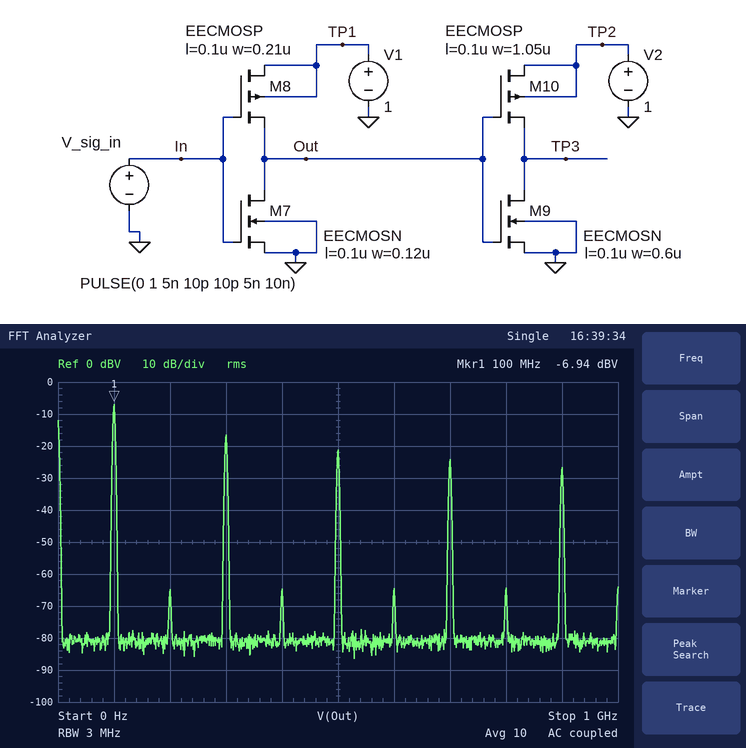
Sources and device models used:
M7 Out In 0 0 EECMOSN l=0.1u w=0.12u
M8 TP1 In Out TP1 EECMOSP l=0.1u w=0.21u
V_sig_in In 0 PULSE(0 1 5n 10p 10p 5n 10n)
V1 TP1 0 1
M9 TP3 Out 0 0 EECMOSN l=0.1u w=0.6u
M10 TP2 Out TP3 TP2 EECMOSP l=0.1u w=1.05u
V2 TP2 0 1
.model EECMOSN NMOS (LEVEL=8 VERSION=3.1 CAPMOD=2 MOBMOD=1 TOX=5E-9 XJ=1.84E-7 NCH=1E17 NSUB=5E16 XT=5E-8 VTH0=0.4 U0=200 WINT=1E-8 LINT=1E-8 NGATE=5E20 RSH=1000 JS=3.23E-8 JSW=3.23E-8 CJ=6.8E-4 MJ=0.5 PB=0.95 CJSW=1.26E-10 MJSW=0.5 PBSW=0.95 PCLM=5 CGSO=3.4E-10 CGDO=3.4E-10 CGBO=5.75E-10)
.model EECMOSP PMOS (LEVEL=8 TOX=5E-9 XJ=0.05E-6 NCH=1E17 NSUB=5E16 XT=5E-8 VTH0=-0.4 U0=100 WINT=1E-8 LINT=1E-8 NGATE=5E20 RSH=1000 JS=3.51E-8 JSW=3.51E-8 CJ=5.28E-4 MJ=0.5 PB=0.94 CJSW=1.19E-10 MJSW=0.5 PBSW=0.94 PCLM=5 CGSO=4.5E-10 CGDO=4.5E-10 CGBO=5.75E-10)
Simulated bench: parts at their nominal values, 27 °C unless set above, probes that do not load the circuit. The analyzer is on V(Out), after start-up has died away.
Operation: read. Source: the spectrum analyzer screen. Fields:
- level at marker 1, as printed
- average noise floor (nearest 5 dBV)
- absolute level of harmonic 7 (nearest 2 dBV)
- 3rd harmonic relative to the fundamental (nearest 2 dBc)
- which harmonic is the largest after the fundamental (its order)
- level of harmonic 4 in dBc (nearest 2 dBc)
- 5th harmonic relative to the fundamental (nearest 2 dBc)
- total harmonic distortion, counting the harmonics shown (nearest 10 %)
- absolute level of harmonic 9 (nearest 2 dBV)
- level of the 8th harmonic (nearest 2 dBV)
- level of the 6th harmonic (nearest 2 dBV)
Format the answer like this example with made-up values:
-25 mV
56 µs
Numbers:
-6.94 dBV
-80 dBV
-24 dBV
-10 dBc
3
-58 dBc
-14 dBc
40 %
-26 dBV
-64 dBV
-64 dBV
